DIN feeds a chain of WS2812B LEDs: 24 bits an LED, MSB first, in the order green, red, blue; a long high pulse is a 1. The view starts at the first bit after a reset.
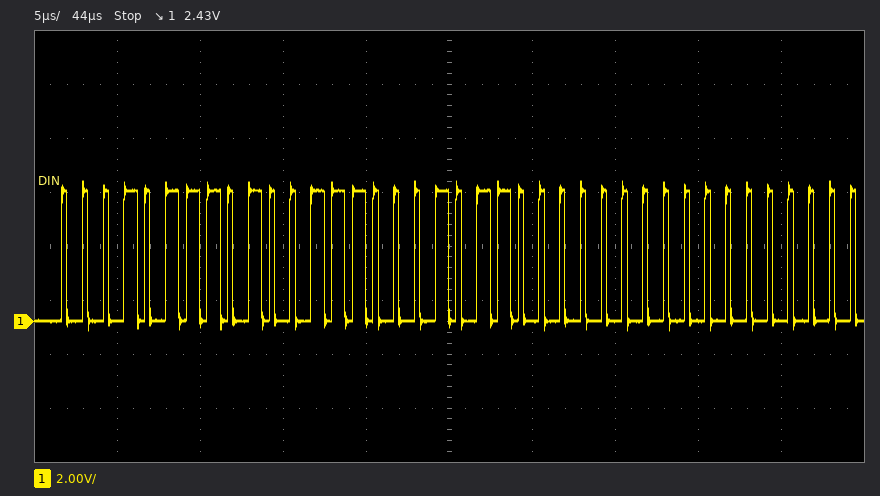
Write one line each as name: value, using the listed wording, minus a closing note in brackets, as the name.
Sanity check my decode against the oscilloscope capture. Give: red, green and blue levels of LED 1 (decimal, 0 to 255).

red, green and blue levels of LED 1: 78, 23, 44
